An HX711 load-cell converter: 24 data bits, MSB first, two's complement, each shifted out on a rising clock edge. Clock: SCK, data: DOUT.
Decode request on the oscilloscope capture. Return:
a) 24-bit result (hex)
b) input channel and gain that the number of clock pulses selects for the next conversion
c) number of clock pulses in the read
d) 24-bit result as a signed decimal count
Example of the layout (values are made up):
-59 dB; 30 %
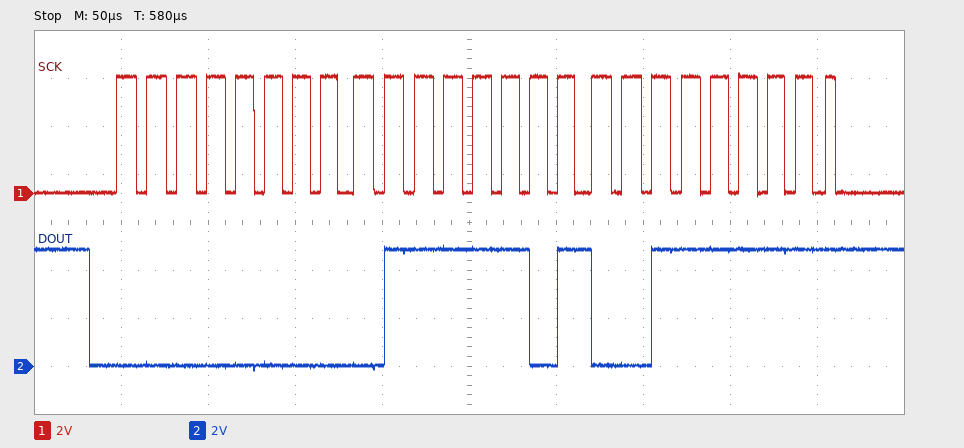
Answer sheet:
0x007D3F; channel A, gain 128; 25; 32063
